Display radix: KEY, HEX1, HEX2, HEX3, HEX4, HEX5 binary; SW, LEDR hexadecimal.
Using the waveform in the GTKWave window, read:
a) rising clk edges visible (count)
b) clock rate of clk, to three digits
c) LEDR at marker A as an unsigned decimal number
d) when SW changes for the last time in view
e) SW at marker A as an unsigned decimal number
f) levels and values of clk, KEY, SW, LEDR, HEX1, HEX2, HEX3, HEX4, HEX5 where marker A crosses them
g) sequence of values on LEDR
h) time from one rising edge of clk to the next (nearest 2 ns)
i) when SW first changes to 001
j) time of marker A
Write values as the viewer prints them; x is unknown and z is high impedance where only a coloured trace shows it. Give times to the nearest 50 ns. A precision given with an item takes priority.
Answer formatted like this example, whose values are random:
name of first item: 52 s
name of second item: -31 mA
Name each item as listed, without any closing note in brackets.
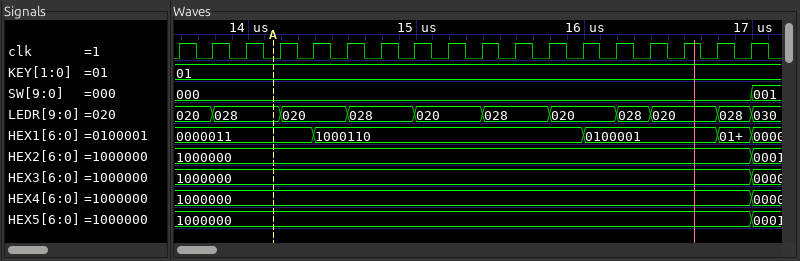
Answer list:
rising clk edges visible: 18
clock rate of clk, to three digits: 5.00 MHz
LEDR at marker A as an unsigned decimal number: 40
when SW changes for the last time in view: 17000 ns
SW at marker A as an unsigned decimal number: 0
levels and values of clk, KEY, SW, LEDR, HEX1, HEX2, HEX3, HEX4, HEX5 where marker A crosses them: clk=0, KEY=01, SW=000, LEDR=028, HEX1=0000011, HEX2=1000000, HEX3=1000000, HEX4=1000000, HEX5=1000000
sequence of values on LEDR: 020, 028, 020, 028, 020, 028, 020, 028, 020, 028, 030
time from one rising edge of clk to the next: 200 ns
when SW first changes to 001: 17000 ns
time of marker A: 14150 ns
